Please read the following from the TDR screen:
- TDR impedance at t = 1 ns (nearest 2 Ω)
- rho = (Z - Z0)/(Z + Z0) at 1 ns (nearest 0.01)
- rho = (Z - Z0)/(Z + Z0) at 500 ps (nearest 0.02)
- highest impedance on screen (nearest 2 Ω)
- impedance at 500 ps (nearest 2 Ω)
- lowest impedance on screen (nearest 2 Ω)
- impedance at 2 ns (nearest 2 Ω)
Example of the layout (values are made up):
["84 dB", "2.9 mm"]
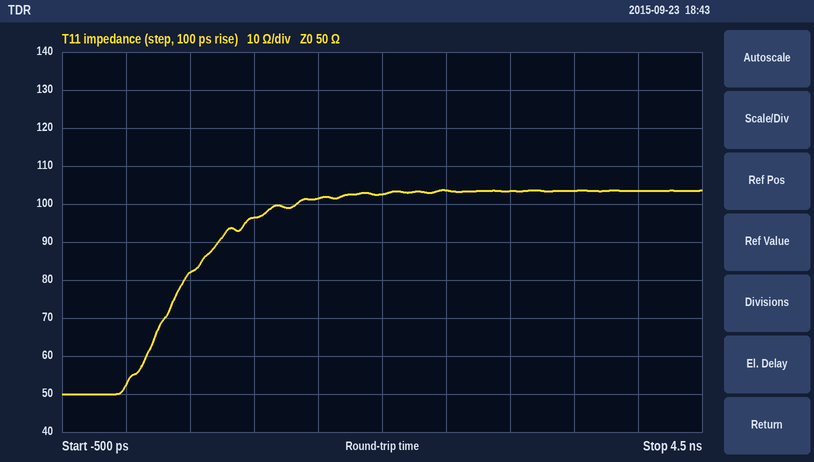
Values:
["96 Ω", "+0.32", "+0.24", "104 Ω", "82 Ω", "50 Ω", "102 Ω"]
